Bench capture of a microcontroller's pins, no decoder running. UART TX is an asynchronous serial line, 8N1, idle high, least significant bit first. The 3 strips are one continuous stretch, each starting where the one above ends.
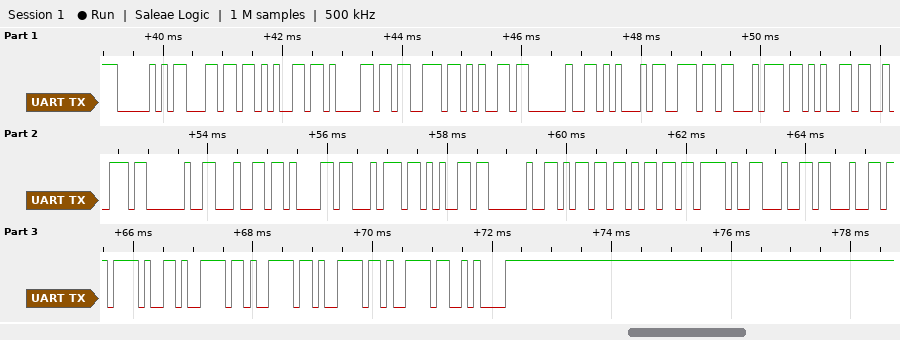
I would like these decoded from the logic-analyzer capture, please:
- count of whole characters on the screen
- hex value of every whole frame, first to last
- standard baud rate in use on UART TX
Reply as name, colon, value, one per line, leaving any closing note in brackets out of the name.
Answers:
count of whole characters on the screen: 29
hex value of every whole frame, first to last: 0x50 0x6C 0x65 0x61 0x73 0x65 0x20 0x45 0x6E 0x74 0x65 0x72 0x20 0x64 0x61 0x74 0x65 0x20 0x6D 0x6D 0x2F 0x64 0x64 0x2F 0x79 0x79 0x79 0x79 0x0A
standard baud rate in use on UART TX: 9600 baud
